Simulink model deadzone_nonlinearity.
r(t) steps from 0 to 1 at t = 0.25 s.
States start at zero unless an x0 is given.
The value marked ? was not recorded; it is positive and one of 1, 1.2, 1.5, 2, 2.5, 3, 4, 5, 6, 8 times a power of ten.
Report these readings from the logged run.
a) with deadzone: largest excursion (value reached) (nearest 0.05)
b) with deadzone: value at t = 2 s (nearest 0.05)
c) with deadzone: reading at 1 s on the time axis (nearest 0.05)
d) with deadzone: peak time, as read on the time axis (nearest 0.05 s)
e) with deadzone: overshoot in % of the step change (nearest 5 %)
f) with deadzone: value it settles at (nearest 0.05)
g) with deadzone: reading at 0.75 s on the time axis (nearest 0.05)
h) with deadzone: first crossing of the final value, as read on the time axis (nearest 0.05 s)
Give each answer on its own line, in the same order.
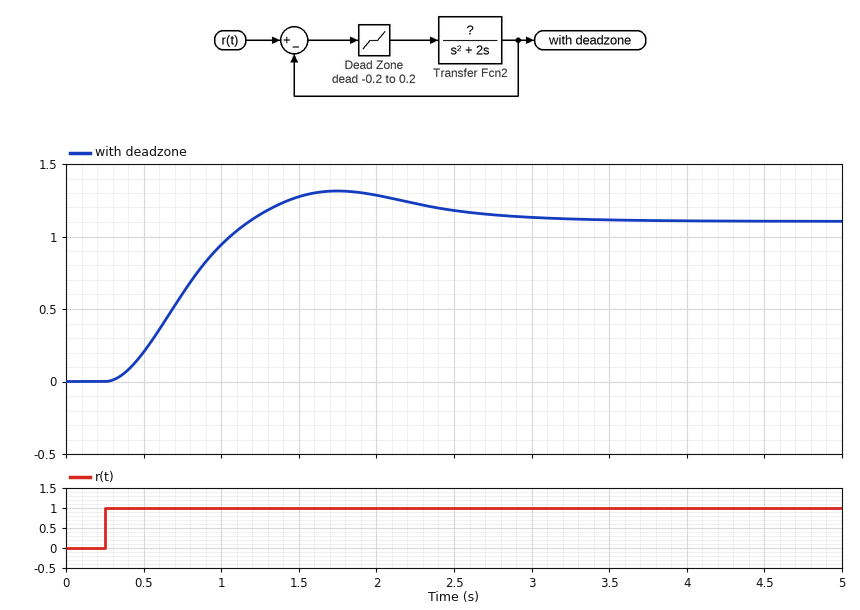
1.30
1.30
0.95
1.75 s
20 %
1.10
0.60
1.20 s
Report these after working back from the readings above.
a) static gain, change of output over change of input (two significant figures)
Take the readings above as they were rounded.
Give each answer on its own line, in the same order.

1.1
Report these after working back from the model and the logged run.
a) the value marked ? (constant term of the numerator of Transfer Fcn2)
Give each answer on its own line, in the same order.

10
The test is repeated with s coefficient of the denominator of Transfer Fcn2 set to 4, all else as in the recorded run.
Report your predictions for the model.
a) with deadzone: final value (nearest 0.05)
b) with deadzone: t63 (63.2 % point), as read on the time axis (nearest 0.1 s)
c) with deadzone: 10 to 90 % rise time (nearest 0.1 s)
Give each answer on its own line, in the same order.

0.90
0.8 s
0.8 s
